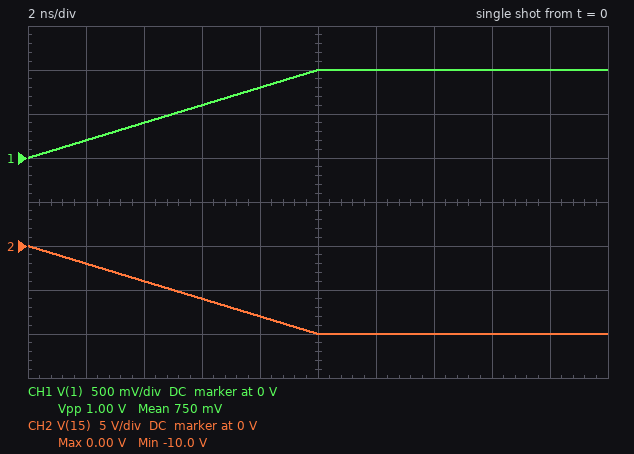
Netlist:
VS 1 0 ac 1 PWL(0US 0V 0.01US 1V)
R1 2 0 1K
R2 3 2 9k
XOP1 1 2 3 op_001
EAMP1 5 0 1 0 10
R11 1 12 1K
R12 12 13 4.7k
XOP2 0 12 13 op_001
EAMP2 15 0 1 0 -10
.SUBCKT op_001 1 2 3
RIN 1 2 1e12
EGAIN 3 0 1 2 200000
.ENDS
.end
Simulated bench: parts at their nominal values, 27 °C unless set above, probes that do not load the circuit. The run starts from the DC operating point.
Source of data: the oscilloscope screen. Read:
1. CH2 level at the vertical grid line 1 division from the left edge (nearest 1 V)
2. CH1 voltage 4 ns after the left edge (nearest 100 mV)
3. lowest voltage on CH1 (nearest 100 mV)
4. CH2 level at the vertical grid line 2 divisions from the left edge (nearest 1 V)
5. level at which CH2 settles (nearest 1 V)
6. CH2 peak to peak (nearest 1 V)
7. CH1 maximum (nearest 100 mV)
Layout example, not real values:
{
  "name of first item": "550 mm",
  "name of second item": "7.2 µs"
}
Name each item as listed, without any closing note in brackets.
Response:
{
  "CH2 level at the vertical grid line 1 division from the left edge": "-2 V",
  "CH1 voltage 4 ns after the left edge": "400 mV",
  "lowest voltage on CH1": "0 V",
  "CH2 level at the vertical grid line 2 divisions from the left edge": "-4 V",
  "level at which CH2 settles": "-10 V",
  "CH2 peak to peak": "10 V",
  "CH1 maximum": "1.0 V"
}
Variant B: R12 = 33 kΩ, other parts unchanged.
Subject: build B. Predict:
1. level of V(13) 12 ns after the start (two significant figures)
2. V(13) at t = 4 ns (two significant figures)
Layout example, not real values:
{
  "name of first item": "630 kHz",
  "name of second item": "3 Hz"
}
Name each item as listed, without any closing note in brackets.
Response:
{
  "level of V(13) 12 ns after the start": "-33 V",
  "V(13) at t = 4 ns": "-13 V"
}
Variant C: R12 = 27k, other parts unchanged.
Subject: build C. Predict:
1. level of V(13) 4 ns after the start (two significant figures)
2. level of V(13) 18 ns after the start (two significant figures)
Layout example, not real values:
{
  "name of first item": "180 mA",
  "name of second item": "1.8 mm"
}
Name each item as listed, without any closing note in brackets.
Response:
{
  "level of V(13) 4 ns after the start": "-11 V",
  "level of V(13) 18 ns after the start": "-27 V"
}
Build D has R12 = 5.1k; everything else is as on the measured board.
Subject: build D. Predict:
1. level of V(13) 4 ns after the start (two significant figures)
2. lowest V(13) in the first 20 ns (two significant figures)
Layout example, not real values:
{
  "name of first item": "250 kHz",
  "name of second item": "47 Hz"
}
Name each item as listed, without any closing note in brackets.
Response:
{
  "level of V(13) 4 ns after the start": "-2.0 V",
  "lowest V(13) in the first 20 ns": "-5.1 V"
}
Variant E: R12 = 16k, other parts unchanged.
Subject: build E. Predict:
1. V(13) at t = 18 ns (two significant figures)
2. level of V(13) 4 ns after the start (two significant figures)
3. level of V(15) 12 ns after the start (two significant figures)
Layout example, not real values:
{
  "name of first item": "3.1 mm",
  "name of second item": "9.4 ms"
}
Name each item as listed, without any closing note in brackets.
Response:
{
  "V(13) at t = 18 ns": "-16 V",
  "level of V(13) 4 ns after the start": "-6.4 V",
  "level of V(15) 12 ns after the start": "-10 V"
}
